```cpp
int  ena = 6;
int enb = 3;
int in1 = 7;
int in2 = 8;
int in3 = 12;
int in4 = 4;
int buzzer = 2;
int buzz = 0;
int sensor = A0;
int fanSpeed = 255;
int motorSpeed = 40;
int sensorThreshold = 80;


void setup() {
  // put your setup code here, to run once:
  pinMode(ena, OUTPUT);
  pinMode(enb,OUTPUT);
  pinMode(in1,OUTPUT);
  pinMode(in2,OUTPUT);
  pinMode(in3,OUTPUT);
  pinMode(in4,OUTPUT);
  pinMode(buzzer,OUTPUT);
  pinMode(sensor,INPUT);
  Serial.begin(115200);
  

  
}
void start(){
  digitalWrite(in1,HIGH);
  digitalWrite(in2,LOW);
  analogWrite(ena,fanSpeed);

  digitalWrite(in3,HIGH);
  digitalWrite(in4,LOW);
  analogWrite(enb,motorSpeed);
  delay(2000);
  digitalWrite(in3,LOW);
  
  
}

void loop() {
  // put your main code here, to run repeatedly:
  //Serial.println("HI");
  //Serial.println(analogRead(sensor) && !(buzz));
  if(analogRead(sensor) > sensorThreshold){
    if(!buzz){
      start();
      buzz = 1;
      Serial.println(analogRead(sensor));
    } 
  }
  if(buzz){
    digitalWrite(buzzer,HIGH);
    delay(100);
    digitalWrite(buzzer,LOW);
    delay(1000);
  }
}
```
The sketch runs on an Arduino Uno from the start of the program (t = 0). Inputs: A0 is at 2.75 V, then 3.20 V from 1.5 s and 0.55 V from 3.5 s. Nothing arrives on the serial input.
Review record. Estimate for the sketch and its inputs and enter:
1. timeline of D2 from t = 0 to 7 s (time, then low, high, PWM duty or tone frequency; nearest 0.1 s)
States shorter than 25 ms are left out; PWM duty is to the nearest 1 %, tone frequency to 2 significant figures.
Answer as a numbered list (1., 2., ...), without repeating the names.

1. 0 s low; 2 s high; 2.1 s low; 3.1 s high; 3.2 s low; 4.2 s high; 4.3 s low; 5.3 s high; 5.4 s low; 6.4 s high; 6.5 s low
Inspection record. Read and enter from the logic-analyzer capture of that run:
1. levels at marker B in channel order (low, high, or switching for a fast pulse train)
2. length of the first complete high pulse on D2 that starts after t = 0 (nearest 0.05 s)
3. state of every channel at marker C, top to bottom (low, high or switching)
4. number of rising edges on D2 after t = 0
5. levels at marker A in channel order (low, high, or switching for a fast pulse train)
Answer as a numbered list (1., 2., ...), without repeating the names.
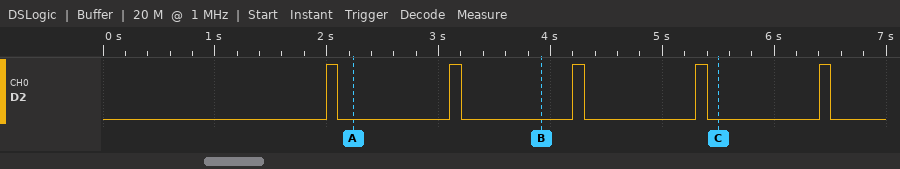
1. D2 low
2. 0.10 s
3. D2 low
4. 5
5. D2 low
